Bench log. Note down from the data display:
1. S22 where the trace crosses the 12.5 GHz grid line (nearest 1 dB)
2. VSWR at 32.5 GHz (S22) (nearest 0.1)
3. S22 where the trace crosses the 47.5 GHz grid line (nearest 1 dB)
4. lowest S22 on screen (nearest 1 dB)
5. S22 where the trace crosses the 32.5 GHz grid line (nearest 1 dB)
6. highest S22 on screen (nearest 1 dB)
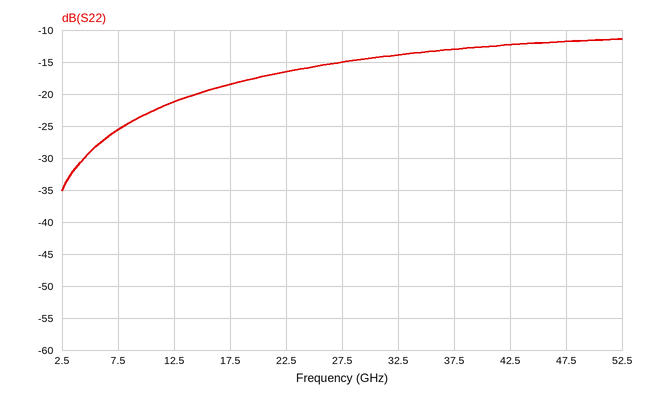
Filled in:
-21 dB
1.5
-12 dB
-35 dB
-14 dB
-11 dB
